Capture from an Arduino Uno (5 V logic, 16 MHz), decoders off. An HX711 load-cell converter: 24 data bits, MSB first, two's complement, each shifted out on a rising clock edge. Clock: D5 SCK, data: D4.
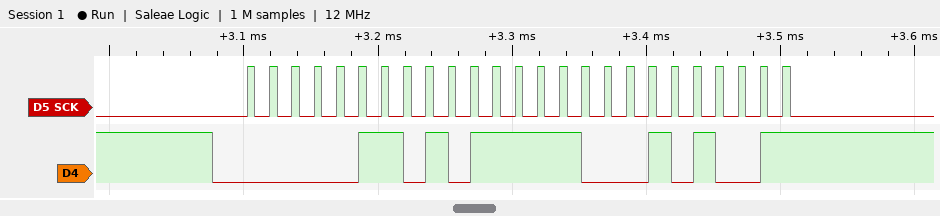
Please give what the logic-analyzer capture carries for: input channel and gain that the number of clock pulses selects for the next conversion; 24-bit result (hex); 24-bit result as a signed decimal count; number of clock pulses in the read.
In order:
channel A, gain 128
0x06BE29
441897
25
